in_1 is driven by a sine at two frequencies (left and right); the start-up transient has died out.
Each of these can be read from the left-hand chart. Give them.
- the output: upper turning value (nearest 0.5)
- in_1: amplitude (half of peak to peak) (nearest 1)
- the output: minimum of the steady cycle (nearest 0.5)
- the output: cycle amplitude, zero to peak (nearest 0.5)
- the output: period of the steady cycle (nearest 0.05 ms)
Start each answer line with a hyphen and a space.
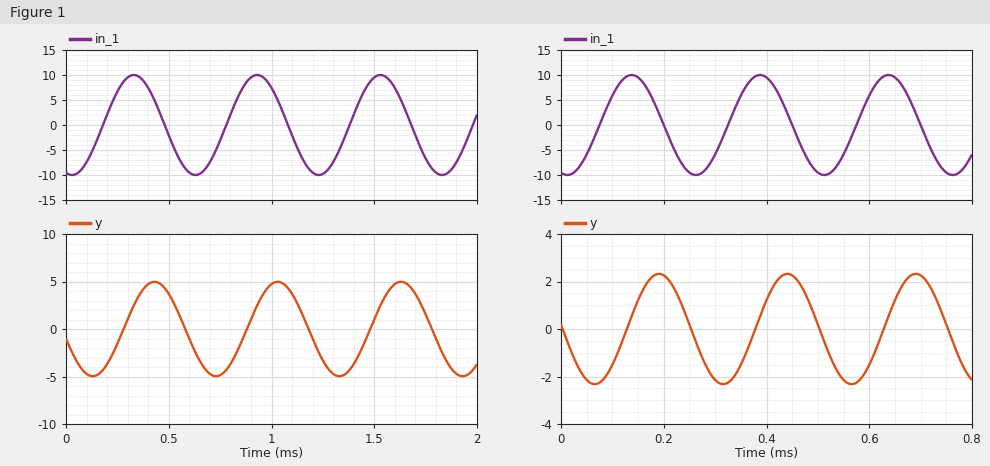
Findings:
- 5.0
- 10
- -5.0
- 5.0
- 0.60 ms
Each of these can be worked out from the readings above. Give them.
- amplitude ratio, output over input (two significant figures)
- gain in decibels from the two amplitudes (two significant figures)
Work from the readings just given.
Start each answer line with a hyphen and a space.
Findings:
- 0.50
- -6.0 dB
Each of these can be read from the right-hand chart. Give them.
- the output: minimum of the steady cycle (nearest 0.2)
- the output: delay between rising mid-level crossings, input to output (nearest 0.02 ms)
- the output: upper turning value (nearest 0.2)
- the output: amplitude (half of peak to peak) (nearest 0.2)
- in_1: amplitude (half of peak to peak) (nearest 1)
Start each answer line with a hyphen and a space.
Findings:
- -2.4
- 0.06 ms
- 2.4
- 2.4
- 10
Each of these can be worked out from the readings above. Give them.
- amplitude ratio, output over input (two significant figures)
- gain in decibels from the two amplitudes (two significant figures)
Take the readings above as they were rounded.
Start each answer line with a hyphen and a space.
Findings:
- 0.24
- -12 dB
